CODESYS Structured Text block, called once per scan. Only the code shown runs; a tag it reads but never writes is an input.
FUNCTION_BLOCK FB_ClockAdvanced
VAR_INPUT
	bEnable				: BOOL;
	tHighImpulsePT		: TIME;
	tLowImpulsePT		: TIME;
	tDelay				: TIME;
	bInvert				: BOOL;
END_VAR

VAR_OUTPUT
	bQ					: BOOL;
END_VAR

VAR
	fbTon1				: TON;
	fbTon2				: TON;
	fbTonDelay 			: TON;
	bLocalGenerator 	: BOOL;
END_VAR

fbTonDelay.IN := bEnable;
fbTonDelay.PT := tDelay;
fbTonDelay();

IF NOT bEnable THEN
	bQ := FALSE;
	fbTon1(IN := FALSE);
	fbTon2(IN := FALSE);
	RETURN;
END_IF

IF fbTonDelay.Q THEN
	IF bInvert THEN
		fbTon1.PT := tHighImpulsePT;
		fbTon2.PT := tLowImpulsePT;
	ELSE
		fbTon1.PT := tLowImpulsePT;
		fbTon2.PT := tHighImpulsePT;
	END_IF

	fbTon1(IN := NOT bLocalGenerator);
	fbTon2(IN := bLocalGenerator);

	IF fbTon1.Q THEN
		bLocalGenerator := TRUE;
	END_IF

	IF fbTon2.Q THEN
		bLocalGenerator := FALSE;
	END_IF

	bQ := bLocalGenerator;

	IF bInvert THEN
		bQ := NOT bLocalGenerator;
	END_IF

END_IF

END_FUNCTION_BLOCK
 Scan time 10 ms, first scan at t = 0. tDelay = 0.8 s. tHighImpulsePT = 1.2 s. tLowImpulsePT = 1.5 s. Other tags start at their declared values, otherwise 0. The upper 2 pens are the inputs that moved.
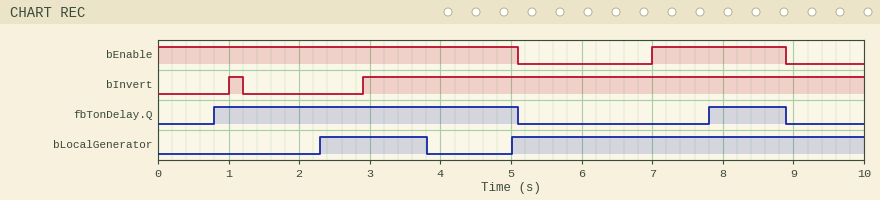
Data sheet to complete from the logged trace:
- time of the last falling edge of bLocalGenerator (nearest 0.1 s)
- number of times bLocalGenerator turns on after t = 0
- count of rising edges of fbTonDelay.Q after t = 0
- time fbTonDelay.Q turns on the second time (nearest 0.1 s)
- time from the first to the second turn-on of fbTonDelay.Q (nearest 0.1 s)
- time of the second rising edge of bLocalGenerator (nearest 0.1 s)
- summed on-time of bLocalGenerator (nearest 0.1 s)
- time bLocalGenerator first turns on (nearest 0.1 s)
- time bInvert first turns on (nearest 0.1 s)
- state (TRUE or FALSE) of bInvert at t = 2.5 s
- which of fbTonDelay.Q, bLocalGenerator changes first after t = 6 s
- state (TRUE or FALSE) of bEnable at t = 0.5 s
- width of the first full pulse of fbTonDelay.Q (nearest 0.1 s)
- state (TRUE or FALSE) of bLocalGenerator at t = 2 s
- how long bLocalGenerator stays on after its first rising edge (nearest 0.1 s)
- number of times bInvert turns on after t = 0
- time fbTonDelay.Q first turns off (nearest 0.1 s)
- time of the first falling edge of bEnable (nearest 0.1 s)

3.8 s
2
2
7.8 s
7.0 s
5.0 s
6.5 s
2.3 s
1.0 s
FALSE
fbTonDelay.Q
TRUE
4.3 s
FALSE
1.5 s
2
5.1 s
5.1 s
